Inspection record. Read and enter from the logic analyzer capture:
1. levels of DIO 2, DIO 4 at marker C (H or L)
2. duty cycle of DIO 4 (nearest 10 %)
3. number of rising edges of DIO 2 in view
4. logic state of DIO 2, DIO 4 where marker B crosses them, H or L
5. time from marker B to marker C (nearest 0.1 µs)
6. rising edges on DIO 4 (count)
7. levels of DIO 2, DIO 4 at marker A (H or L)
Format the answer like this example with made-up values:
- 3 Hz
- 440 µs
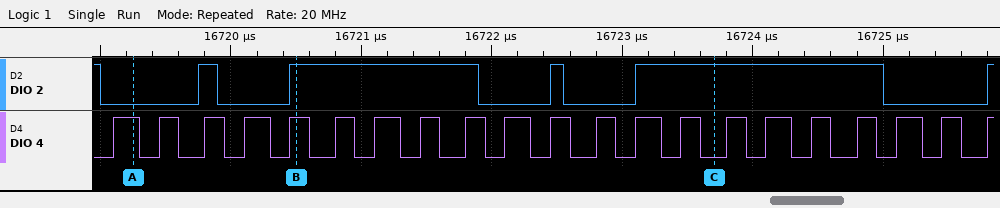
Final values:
- DIO 2=H, DIO 4=L
- 50 %
- 5
- DIO 2=H, DIO 4=H
- 3.2 µs
- 21
- DIO 2=L, DIO 4=H
